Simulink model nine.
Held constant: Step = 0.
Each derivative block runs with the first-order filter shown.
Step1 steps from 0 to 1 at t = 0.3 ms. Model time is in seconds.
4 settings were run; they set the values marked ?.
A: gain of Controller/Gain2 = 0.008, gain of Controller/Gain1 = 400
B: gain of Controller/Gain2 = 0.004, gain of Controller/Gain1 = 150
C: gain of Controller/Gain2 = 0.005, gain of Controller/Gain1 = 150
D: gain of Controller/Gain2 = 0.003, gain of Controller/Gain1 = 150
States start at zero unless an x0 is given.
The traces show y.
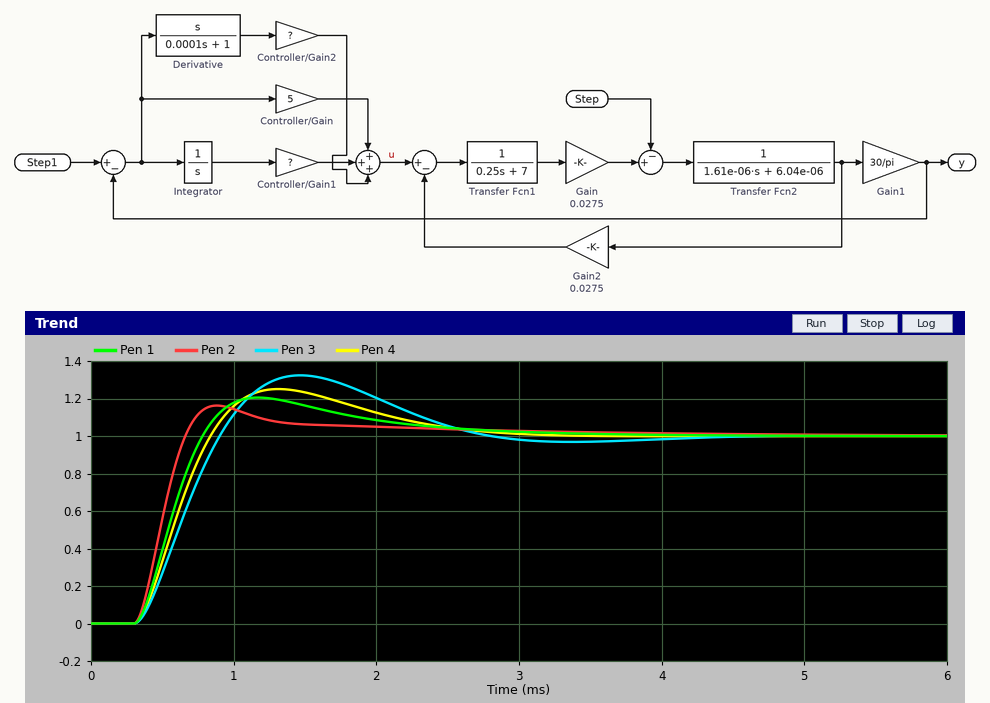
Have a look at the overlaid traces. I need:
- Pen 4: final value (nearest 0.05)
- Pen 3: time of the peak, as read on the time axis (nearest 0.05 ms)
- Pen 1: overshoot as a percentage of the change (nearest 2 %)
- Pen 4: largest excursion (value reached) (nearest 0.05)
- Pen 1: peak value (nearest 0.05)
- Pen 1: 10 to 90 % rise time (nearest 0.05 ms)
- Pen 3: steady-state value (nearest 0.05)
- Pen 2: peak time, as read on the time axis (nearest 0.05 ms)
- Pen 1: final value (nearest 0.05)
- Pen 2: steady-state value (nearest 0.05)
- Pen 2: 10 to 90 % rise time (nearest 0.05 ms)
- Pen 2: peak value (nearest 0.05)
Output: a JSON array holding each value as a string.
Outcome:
["1.00", "1.45 ms", "20 %", "1.25", "1.20", "0.35 ms", "1.00", "0.90 ms", "1.00", "1.00", "0.25 ms", "1.15"]
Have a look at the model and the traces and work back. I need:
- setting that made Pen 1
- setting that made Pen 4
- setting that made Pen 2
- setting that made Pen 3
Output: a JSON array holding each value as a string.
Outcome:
["C", "B", "A", "D"]
